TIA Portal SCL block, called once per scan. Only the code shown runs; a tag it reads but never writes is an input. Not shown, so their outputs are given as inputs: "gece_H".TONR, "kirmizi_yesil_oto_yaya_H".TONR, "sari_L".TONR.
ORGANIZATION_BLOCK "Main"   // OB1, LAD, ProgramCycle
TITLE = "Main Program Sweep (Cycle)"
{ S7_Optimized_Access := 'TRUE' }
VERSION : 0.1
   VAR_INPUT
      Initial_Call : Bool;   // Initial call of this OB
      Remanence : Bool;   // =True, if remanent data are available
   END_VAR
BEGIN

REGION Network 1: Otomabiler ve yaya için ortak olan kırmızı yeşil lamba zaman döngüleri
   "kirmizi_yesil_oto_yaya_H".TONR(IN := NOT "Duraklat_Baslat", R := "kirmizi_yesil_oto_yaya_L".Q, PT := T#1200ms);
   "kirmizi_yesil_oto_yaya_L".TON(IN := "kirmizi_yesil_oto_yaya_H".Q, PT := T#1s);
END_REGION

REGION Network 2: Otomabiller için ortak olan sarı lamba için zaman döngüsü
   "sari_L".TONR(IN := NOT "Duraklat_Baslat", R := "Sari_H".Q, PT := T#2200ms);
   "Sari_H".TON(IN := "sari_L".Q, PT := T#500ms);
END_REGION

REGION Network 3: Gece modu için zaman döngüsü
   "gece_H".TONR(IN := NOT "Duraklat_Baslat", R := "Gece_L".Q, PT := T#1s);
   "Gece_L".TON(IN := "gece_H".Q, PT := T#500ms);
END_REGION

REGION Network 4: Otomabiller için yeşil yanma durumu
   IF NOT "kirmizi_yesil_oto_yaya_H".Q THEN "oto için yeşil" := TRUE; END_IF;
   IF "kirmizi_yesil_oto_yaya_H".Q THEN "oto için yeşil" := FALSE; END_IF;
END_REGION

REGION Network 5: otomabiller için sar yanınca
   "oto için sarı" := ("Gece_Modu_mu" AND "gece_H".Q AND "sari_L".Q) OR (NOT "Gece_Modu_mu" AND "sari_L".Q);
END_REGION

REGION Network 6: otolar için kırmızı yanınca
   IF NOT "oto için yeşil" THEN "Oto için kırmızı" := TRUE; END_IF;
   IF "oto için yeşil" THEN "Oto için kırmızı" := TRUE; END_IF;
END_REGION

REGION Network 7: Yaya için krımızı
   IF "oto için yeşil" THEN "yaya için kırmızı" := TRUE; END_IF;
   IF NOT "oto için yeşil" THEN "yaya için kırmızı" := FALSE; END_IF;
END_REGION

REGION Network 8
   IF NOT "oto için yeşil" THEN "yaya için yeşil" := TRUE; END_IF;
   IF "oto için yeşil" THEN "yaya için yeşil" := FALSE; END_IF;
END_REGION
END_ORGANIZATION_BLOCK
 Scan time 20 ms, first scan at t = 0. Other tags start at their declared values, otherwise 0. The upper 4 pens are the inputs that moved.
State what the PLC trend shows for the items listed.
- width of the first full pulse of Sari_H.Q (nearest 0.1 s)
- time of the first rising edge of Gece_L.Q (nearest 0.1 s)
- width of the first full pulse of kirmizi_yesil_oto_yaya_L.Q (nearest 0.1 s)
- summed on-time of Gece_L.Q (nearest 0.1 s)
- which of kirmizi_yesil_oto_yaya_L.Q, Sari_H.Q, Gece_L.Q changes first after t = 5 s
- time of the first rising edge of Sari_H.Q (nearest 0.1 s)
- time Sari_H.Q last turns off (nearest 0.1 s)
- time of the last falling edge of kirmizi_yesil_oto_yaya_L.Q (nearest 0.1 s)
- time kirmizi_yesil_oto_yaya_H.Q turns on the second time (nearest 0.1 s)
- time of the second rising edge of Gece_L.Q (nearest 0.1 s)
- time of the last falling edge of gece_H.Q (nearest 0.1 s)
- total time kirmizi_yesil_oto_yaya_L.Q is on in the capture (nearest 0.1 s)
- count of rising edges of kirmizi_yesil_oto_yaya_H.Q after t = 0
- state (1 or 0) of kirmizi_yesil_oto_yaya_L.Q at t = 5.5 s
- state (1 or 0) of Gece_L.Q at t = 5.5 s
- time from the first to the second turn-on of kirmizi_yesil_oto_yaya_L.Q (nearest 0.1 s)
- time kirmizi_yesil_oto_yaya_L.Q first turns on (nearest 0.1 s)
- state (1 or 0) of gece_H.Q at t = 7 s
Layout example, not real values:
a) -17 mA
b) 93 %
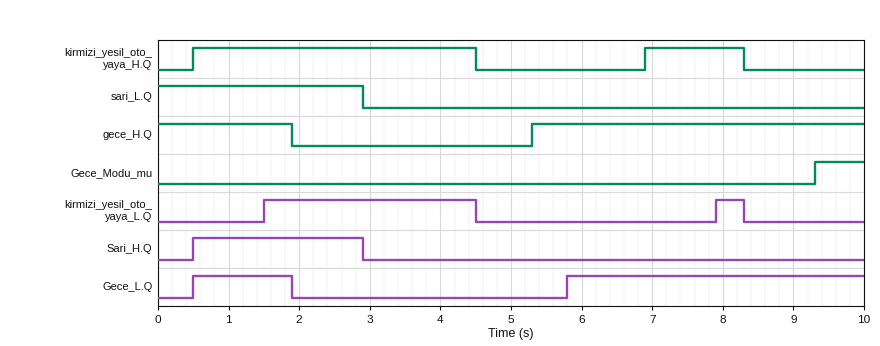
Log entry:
a) 2.4 s
b) 0.5 s
c) 3.0 s
d) 5.6 s
e) Gece_L.Q
f) 0.5 s
g) 2.9 s
h) 8.3 s
i) 6.9 s
j) 5.8 s
k) 1.9 s
l) 3.4 s
m) 2
n) 0
o) 0
p) 6.4 s
q) 1.5 s
r) 1
